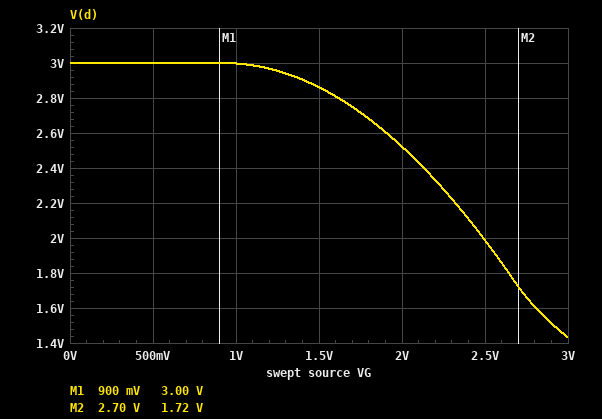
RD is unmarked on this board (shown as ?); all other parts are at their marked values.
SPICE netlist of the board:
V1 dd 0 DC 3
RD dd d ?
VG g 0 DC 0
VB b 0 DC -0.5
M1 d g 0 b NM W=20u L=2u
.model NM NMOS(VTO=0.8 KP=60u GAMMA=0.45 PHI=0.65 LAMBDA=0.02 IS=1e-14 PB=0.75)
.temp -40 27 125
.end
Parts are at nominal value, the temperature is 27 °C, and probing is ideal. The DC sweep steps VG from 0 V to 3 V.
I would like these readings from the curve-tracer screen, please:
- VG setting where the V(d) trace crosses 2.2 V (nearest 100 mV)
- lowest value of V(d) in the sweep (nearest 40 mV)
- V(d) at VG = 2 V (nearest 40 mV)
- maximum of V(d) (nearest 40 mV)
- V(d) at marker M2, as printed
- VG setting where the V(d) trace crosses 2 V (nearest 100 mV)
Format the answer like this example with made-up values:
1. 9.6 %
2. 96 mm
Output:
1. 2.3 V
2. 1.44 V
3. 2.52 V
4. 3.00 V
5. 1.72 V
6. 2.5 V
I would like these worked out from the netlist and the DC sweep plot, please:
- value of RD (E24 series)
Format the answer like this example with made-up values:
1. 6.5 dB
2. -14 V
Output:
1. 1.3 kΩ
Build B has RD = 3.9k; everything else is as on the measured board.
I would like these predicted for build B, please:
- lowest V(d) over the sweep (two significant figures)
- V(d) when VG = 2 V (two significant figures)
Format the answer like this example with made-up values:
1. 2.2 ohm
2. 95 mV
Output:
1. 570 mV
2. 1.6 V
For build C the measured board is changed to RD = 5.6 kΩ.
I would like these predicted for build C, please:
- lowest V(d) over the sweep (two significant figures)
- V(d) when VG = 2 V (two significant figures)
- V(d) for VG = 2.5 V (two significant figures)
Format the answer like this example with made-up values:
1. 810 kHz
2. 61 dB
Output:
1. 410 mV
2. 1.0 V
3. 550 mV
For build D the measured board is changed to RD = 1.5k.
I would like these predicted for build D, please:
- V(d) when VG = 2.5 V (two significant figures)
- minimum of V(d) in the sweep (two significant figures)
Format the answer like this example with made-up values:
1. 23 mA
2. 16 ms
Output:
1. 1.8 V
2. 1.3 V
